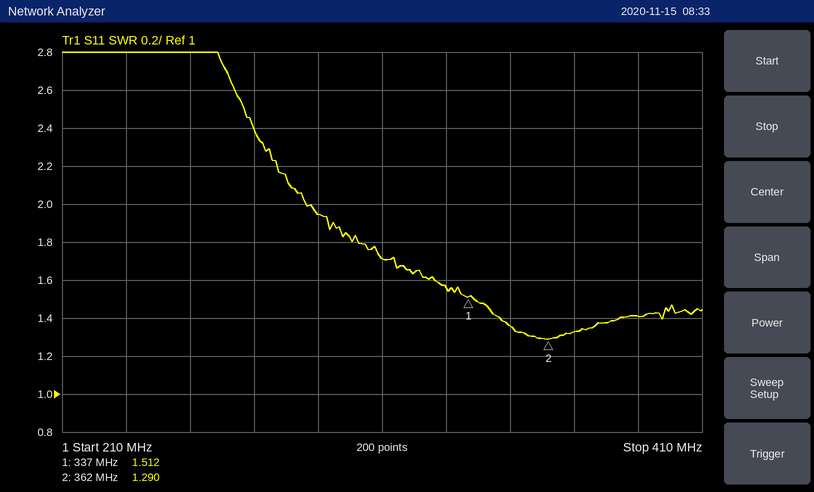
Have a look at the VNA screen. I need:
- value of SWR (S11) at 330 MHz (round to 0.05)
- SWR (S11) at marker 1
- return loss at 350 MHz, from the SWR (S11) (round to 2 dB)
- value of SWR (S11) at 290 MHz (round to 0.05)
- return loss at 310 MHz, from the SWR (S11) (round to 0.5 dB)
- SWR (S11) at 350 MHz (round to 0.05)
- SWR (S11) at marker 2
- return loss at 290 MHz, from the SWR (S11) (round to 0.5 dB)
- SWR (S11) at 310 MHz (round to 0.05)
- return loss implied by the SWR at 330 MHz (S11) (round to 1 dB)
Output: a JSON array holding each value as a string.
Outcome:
["1.55", "1.512", "16 dB", "1.95", "11.5 dB", "1.35", "1.290", "10.0 dB", "1.70", "13 dB"]
